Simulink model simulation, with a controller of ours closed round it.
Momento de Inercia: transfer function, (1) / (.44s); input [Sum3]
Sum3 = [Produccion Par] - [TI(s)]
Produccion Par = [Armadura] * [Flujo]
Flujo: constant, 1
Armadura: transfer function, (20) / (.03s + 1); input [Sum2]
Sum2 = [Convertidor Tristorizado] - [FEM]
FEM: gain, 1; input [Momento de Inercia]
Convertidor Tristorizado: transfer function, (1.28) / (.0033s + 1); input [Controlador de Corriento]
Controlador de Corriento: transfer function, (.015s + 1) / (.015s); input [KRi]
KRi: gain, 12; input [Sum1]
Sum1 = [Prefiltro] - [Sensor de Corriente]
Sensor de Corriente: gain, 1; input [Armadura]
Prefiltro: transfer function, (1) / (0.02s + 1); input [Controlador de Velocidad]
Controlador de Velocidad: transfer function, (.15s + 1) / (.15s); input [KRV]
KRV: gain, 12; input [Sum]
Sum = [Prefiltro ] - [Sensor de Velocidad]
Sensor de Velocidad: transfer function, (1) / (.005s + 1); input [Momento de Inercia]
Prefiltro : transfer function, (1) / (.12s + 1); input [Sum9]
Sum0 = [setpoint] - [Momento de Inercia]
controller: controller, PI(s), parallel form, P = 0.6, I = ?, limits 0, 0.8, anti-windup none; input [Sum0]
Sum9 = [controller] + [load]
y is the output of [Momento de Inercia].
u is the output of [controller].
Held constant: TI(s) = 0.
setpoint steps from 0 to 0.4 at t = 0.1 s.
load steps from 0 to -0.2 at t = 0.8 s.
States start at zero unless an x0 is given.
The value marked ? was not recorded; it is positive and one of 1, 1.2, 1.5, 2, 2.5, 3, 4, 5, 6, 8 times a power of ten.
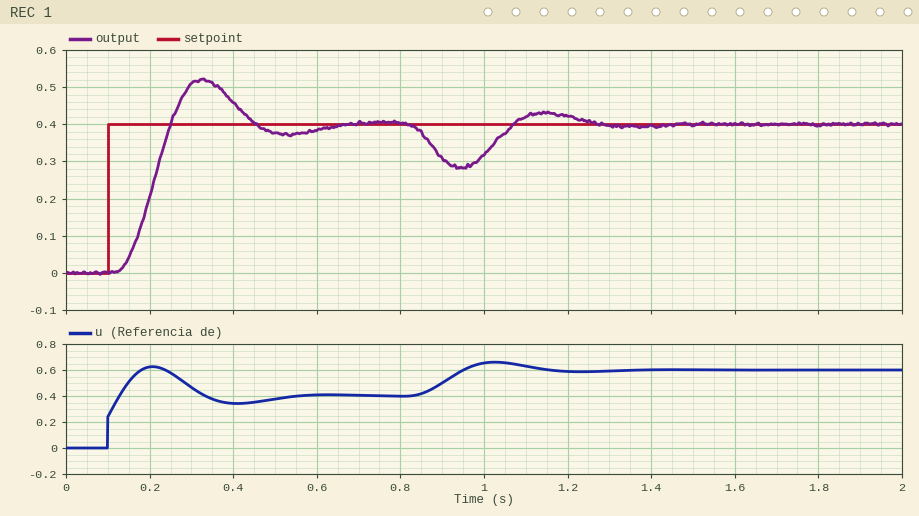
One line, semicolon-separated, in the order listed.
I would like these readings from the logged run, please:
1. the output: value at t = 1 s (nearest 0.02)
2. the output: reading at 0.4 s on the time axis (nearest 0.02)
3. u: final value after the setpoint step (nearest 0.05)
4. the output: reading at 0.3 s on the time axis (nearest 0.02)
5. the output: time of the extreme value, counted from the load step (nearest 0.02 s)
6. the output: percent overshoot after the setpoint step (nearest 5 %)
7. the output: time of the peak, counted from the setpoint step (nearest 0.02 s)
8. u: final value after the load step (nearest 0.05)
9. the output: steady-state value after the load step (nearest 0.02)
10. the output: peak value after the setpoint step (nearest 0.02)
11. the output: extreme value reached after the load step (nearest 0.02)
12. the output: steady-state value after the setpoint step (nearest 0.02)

0.32; 0.46; 0.40; 0.50; 0.14 s; 30 %; 0.22 s; 0.60; 0.40; 0.52; 0.28; 0.40
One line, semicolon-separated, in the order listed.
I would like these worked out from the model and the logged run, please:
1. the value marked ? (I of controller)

15
